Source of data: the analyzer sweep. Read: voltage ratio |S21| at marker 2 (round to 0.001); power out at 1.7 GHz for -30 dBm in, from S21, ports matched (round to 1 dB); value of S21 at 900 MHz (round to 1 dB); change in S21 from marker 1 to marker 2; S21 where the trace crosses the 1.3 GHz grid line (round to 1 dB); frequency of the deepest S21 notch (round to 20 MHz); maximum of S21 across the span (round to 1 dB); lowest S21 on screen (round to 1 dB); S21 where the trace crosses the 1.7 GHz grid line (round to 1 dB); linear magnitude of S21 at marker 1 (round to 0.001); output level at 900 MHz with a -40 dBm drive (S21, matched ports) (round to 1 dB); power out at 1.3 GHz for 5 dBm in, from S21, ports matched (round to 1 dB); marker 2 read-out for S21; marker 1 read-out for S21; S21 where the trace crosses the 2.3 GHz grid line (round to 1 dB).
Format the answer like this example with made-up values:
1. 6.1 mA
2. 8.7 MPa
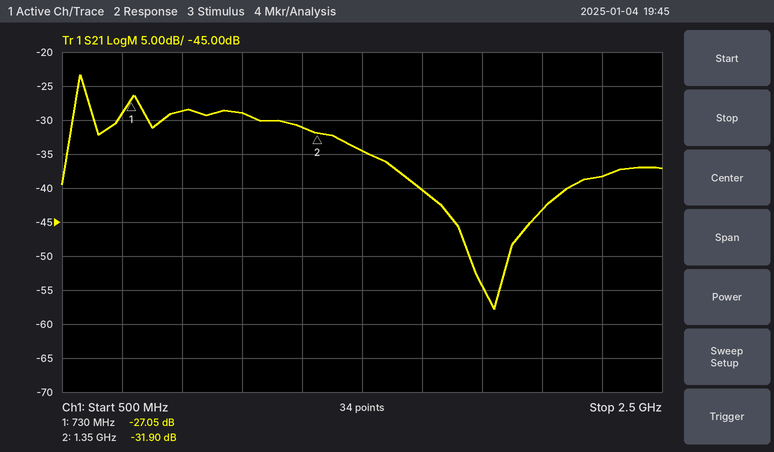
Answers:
1. 0.025
2. -70 dBm
3. -29 dB
4. -4.85 dB
5. -31 dB
6. 1.94 GHz
7. -23 dB
8. -58 dB
9. -40 dB
10. 0.044
11. -69 dBm
12. -26 dBm
13. -31.90 dB
14. -27.05 dB
15. -38 dB
